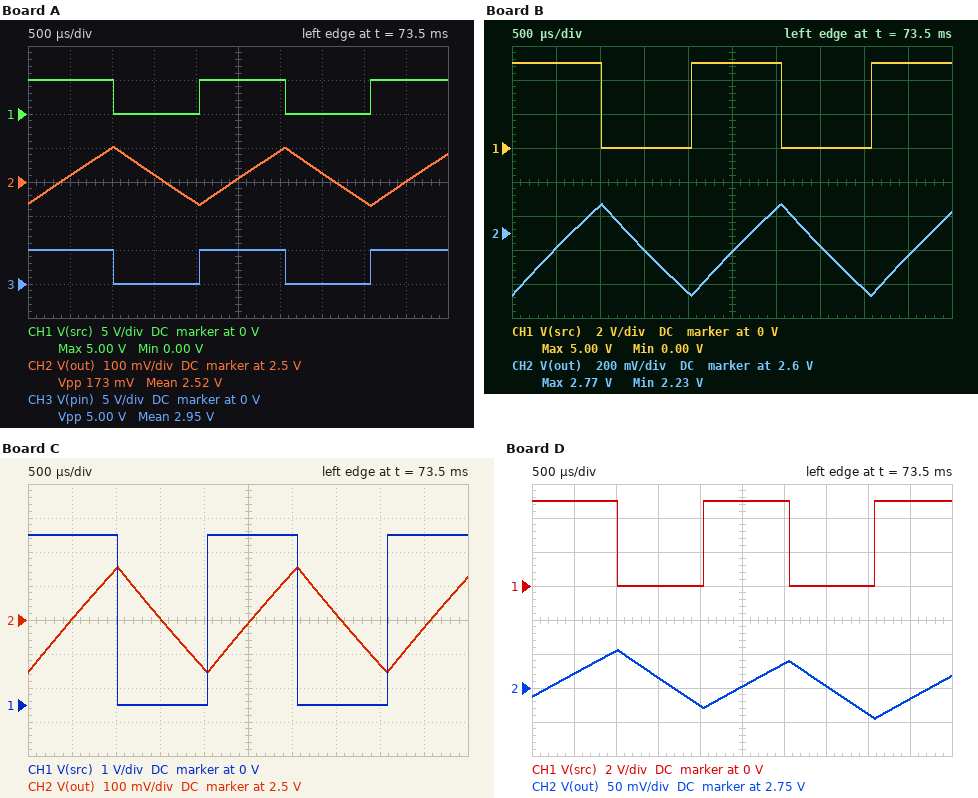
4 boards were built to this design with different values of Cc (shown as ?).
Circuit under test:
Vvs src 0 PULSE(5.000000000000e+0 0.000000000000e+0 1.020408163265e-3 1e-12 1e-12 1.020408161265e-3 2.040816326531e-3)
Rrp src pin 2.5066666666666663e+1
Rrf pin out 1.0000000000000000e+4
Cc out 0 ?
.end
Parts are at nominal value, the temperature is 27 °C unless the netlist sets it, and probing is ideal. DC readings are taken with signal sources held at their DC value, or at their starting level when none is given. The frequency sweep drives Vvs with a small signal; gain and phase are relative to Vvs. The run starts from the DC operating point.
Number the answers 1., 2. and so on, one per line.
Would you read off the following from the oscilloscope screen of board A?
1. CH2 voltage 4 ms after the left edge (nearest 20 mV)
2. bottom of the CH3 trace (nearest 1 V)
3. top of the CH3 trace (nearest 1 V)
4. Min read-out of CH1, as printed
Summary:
1. 2.44 V
2. 0 V
3. 5 V
4. 0.00 V
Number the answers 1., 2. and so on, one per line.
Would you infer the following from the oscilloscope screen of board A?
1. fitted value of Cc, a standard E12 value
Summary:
1. 1.5 µF
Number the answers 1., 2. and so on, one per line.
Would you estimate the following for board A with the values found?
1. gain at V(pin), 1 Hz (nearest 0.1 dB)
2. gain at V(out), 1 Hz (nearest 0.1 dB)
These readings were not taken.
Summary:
1. 0 dB
2. 0 dB
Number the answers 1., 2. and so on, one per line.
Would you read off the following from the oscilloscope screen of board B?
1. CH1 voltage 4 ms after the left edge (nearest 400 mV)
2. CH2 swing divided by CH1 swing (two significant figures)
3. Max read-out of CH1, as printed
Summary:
1. 0 V
2. 0.11
3. 5.00 V
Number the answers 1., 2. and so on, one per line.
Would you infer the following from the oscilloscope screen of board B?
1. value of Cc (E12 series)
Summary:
1. 470 nF
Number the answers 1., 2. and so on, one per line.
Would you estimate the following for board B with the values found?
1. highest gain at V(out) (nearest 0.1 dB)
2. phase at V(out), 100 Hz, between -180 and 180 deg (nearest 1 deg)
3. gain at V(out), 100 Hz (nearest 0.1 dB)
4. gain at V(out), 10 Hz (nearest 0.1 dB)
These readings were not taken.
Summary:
1. 0 dB
2. -71 deg
3. -9.9 dB
4. -0.4 dB
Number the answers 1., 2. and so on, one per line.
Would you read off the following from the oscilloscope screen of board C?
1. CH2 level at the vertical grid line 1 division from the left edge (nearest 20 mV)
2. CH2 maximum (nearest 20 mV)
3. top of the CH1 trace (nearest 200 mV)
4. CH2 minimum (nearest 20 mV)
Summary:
1. 2.50 V
2. 2.66 V
3. 5.0 V
4. 2.34 V
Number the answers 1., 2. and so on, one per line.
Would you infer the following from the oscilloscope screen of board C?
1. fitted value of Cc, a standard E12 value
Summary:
1. 820 nF
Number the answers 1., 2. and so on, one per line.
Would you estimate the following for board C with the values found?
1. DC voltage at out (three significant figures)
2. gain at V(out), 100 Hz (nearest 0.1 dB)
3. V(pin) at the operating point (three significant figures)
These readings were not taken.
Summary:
1. 5.00 V
2. -14.4 dB
3. 5.00 V
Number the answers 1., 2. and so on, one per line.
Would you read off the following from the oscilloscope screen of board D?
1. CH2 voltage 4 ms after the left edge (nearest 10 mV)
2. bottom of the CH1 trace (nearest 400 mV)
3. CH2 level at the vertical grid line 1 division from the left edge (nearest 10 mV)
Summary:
1. 2.71 V
2. 0 V
3. 2.77 V
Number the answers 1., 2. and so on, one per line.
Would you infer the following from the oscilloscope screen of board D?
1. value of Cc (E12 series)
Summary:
1. 3.3 µF
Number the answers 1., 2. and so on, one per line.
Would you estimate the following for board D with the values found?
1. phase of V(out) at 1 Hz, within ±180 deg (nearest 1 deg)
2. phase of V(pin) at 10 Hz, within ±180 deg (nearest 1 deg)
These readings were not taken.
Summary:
1. -12 deg
2. 0 deg
